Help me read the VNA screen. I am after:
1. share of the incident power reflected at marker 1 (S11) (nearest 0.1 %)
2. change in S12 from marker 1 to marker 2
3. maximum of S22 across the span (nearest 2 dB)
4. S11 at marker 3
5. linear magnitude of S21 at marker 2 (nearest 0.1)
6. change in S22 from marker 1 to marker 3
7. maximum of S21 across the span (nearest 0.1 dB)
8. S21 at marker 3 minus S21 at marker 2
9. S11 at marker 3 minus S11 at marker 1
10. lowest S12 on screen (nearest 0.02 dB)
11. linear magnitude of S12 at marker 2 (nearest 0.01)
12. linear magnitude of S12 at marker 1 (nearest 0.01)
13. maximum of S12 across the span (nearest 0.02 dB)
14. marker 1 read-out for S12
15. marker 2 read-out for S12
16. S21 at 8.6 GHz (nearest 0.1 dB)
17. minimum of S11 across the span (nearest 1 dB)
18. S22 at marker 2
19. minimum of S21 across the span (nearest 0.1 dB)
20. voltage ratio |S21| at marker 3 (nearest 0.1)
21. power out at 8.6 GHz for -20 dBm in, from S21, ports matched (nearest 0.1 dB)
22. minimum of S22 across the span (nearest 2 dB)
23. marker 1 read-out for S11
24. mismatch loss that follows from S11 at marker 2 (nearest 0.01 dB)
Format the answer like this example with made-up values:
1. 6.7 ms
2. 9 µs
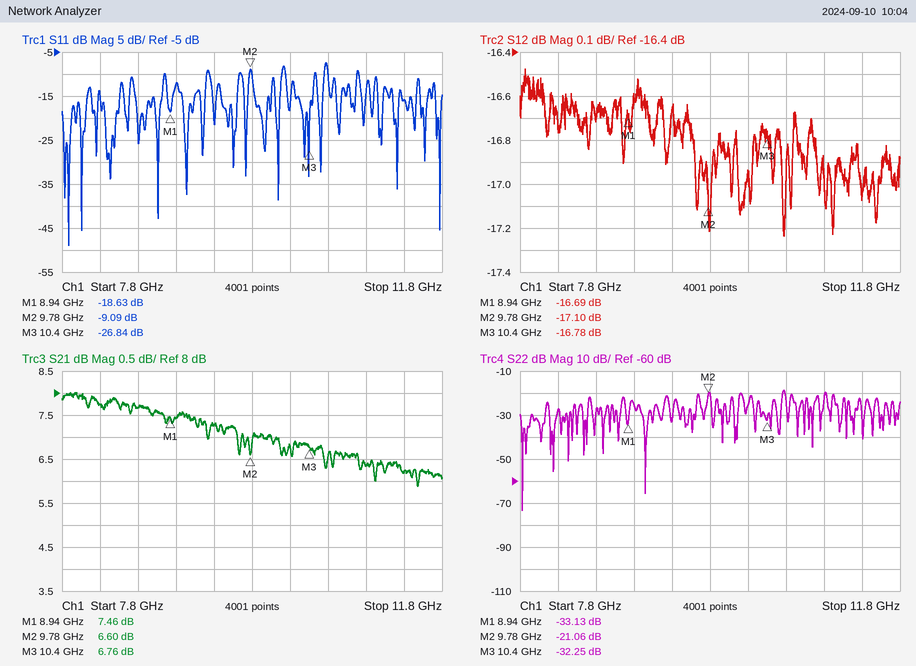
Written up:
1. 1.4 %
2. -0.41 dB
3. -18 dB
4. -26.84 dB
5. 2.1
6. 0.88 dB
7. 8.0 dB
8. 0.16 dB
9. -8.21 dB
10. -17.24 dB
11. 0.14
12. 0.15
13. -16.48 dB
14. -16.69 dB
15. -17.10 dB
16. 7.7 dB
17. -49 dB
18. -21.06 dB
19. 5.9 dB
20. 2.2
21. -12.3 dBm
22. -74 dB
23. -18.63 dB
24. 0.57 dB
